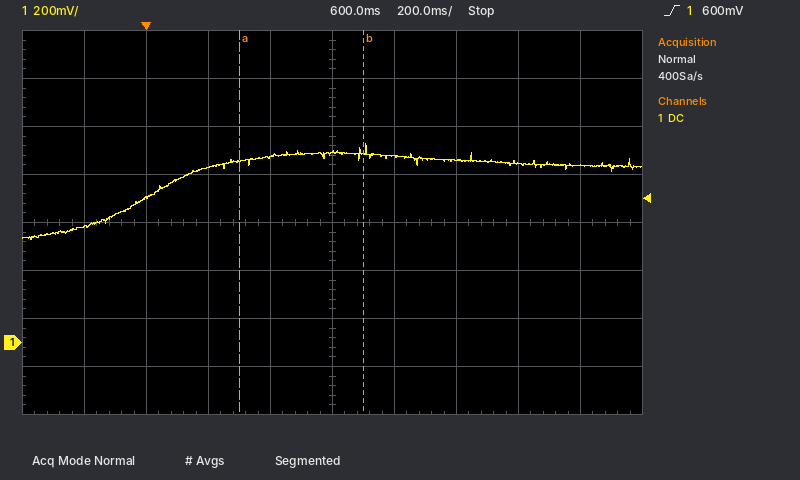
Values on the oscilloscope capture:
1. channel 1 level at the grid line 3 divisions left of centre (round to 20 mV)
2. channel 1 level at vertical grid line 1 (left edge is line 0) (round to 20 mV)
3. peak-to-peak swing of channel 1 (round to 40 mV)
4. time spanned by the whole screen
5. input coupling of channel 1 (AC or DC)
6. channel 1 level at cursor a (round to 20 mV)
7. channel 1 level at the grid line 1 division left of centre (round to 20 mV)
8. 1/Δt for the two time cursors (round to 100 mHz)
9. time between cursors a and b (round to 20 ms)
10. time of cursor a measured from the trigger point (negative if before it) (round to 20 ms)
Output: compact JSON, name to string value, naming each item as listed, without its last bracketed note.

{"channel 1 level at the grid line 3 divisions left of centre": "600 mV", "channel 1 level at vertical grid line 1 (left edge is line 0)": "480 mV", "peak-to-peak swing of channel 1": "400 mV", "time spanned by the whole screen": "2 s", "input coupling of channel 1": "DC", "channel 1 level at cursor a": "760 mV", "channel 1 level at the grid line 1 division left of centre": "780 mV", "1/Δt for the two time cursors": "2.5 Hz", "time between cursors a and b": "400 ms", "time of cursor a measured from the trigger point (negative if before it)": "+300 ms"}
